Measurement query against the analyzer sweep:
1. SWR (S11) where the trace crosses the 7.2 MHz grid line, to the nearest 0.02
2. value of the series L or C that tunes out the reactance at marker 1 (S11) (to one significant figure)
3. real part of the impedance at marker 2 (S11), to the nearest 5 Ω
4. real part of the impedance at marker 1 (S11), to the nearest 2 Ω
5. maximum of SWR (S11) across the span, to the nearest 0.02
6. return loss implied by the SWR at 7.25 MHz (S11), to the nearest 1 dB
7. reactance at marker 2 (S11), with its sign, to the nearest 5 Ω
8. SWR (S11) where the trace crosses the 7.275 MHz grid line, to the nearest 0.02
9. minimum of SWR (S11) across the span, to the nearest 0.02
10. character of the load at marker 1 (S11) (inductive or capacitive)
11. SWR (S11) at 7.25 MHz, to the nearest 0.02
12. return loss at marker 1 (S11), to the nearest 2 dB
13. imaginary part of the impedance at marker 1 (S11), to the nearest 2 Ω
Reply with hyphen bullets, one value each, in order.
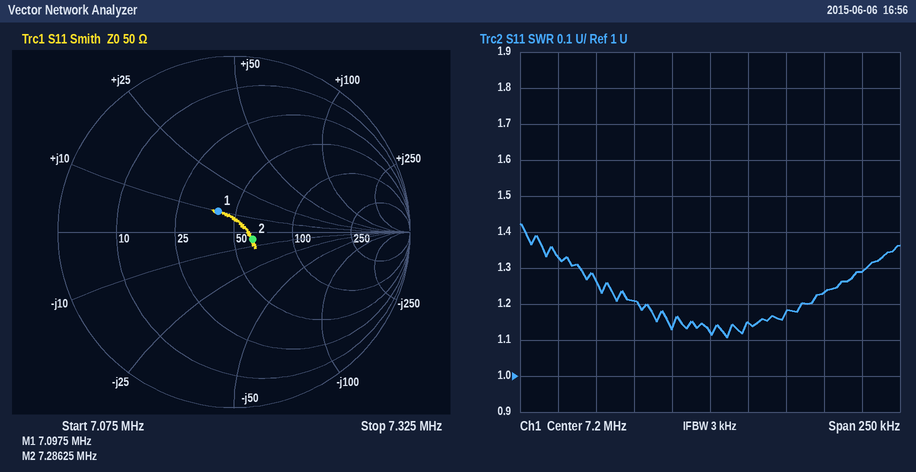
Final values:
- 1.12
- 2 nF
- 60 Ω
- 40 Ω
- 1.42
- 22 dB
- -5 Ω
- 1.24
- 1.10
- inductive
- 1.18
- 16 dB
- +10 Ω
